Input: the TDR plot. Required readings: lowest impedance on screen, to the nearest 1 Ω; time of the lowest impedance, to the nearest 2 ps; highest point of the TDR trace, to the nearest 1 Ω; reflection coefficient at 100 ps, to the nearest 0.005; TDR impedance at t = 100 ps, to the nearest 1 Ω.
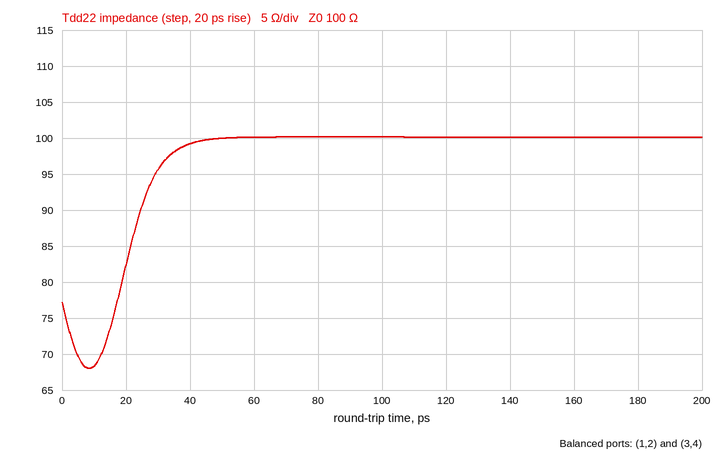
68 Ω
8 ps
100 Ω
0.000
100 Ω
